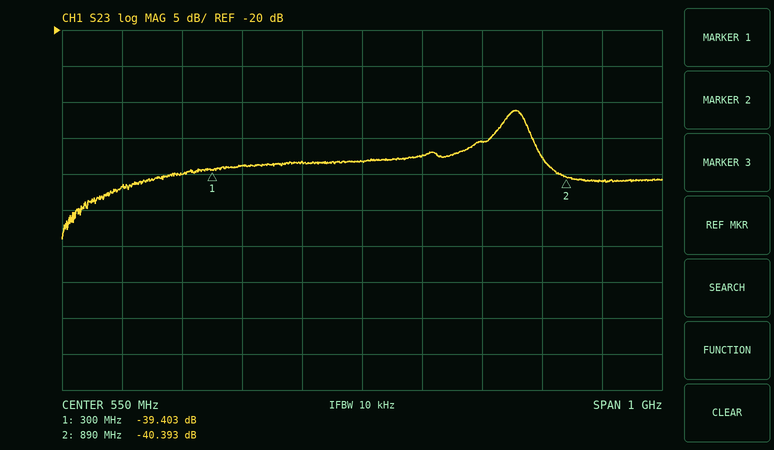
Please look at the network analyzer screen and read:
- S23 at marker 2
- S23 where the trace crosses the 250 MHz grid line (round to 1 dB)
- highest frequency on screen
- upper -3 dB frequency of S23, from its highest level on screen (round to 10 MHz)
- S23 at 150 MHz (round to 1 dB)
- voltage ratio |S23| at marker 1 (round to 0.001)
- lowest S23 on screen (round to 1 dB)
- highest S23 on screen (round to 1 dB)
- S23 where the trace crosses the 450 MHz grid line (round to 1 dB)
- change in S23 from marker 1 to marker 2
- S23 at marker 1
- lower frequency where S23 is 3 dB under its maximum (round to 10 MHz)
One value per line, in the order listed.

-40.393 dB
-40 dB
1.05 GHz
830 MHz
-42 dB
0.011
-49 dB
-31 dB
-38 dB
-0.990 dB
-39.403 dB
770 MHz
